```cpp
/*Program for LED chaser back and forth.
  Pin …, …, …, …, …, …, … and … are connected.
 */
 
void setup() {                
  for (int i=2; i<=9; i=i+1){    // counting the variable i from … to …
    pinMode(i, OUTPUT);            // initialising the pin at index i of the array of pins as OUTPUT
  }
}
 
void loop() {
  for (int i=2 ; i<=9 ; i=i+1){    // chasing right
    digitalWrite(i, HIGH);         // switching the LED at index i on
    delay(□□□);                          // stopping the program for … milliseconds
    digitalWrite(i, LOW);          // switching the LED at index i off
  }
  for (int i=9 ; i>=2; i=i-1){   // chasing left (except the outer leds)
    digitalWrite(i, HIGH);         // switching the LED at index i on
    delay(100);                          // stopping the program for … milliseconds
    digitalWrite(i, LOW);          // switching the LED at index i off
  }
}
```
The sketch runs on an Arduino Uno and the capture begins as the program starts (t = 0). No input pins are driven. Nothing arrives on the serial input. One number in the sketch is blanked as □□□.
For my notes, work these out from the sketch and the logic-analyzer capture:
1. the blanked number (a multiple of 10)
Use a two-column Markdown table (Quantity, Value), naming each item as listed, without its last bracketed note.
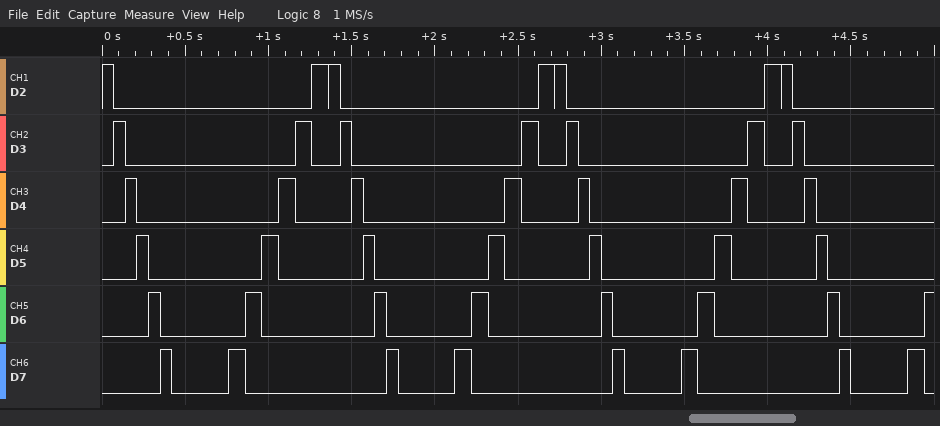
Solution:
| Quantity | Value |
|---|---|
| the blanked number | 70 |
